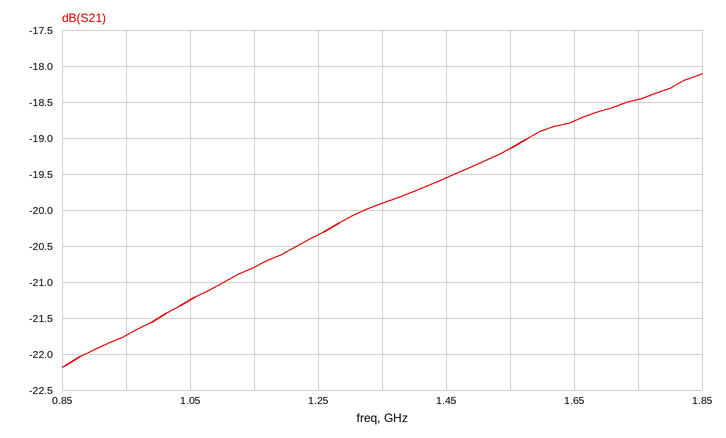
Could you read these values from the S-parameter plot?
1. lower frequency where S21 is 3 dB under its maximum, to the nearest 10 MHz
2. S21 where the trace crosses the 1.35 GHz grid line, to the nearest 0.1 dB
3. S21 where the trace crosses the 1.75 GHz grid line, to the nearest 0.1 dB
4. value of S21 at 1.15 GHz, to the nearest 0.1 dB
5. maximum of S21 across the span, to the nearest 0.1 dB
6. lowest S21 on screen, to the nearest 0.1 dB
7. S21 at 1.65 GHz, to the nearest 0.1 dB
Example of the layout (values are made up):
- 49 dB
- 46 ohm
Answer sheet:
- 1.08 GHz
- -19.9 dB
- -18.5 dB
- -20.8 dB
- -18.1 dB
- -22.2 dB
- -18.8 dB
